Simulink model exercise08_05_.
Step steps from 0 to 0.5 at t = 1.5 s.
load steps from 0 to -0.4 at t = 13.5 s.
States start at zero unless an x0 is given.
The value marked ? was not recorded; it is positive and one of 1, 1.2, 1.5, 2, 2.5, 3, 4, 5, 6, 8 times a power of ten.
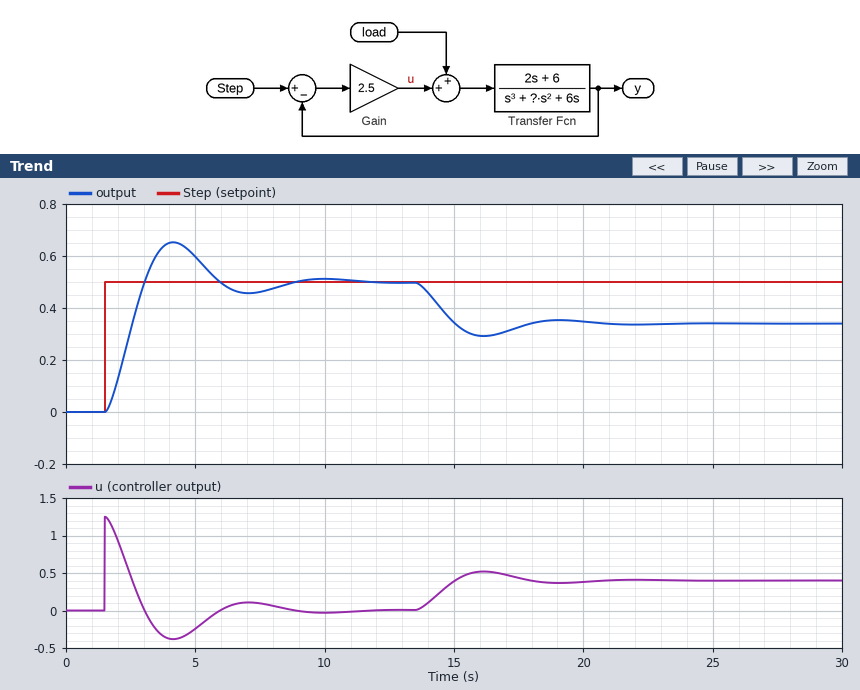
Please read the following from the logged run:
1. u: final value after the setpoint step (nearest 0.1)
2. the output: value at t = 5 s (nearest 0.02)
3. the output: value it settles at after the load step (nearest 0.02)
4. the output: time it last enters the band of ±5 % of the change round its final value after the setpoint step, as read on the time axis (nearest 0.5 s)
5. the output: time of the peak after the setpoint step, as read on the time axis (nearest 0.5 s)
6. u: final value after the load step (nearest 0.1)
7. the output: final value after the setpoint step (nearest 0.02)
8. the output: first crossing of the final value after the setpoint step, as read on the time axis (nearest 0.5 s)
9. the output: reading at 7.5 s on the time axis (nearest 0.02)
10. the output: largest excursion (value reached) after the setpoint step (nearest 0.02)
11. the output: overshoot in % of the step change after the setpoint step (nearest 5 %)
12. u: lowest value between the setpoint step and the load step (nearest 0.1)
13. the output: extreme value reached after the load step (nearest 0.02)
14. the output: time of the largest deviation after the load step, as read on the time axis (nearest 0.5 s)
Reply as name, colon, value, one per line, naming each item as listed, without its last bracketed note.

u: final value after the setpoint step: 0.0
the output: value at t = 5 s: 0.60
the output: value it settles at after the load step: 0.34
the output: time it last enters the band of ±5 % of the change round its final value after the setpoint step, as read on the time axis: 8.0 s
the output: time of the peak after the setpoint step, as read on the time axis: 4.0 s
u: final value after the load step: 0.4
the output: final value after the setpoint step: 0.50
the output: first crossing of the final value after the setpoint step, as read on the time axis: 3.0 s
the output: reading at 7.5 s on the time axis: 0.46
the output: largest excursion (value reached) after the setpoint step: 0.66
the output: overshoot in % of the step change after the setpoint step: 30 %
u: lowest value between the setpoint step and the load step: -0.4
the output: extreme value reached after the load step: 0.30
the output: time of the largest deviation after the load step, as read on the time axis: 16.0 s
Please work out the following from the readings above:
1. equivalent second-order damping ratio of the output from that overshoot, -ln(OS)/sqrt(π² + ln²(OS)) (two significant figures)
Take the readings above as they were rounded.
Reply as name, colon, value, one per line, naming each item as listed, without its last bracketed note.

equivalent second-order damping ratio of the output from that overshoot, -ln(OS)/sqrt(π² + ln²(OS)): 0.36
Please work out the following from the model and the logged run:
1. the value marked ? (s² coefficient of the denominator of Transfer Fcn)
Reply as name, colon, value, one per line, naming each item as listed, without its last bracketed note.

the value marked ?: 12
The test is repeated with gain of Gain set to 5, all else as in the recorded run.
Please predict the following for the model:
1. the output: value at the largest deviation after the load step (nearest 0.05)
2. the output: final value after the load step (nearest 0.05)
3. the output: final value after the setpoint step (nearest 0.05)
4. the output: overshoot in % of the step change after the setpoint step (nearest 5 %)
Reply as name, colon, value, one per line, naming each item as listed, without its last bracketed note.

the output: value at the largest deviation after the load step: 0.40
the output: final value after the load step: 0.40
the output: final value after the setpoint step: 0.50
the output: overshoot in % of the step change after the setpoint step: 35 %
